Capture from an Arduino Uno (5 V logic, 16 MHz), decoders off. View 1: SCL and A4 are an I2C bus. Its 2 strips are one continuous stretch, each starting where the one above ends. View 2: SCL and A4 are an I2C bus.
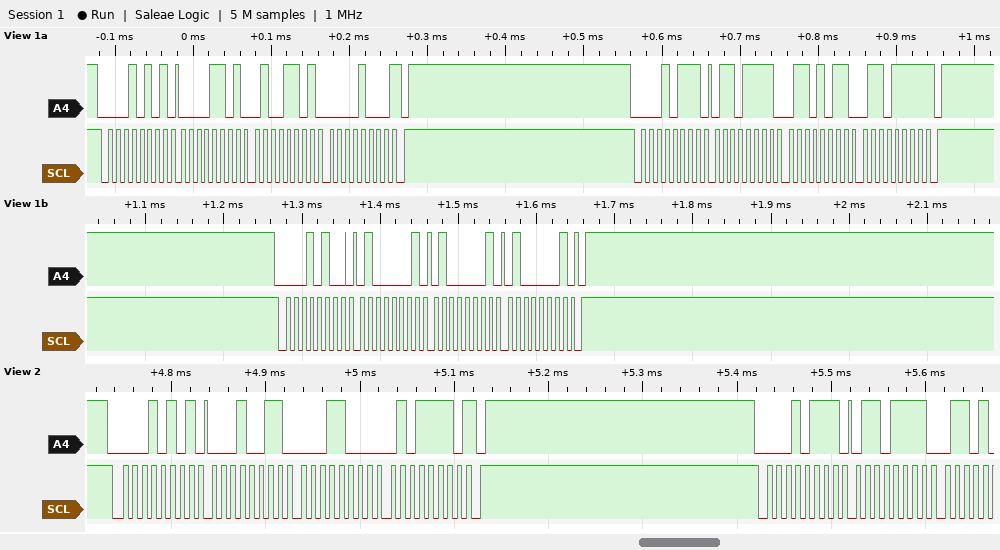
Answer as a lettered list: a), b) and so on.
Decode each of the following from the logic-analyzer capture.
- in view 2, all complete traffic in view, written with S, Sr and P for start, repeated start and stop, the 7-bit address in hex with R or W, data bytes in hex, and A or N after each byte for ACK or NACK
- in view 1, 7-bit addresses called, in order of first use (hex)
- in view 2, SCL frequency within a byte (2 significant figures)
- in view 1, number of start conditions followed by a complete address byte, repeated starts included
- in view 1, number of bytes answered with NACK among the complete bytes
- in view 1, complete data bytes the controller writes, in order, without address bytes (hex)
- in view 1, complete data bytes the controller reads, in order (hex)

a) S 0AR A 13 A 18 A 5E N P S 0BR A 6F A
b) 0x0A 0x0B
c) 100 kHz
d) 3
e) 2
f) 41 41 41
g) 0D 4D 08 6F 6B 6F
